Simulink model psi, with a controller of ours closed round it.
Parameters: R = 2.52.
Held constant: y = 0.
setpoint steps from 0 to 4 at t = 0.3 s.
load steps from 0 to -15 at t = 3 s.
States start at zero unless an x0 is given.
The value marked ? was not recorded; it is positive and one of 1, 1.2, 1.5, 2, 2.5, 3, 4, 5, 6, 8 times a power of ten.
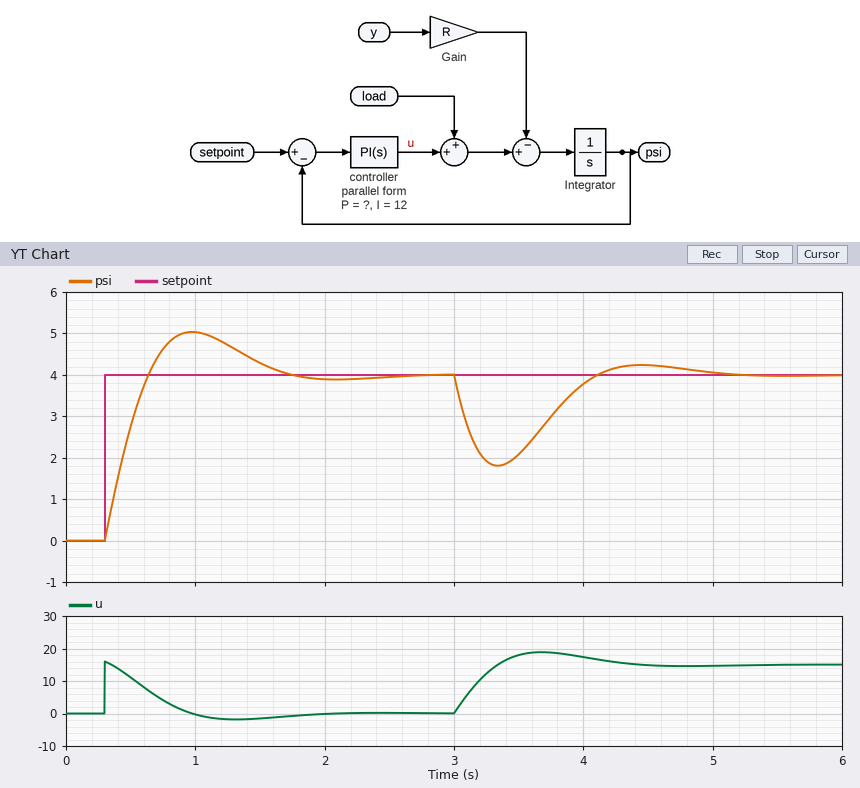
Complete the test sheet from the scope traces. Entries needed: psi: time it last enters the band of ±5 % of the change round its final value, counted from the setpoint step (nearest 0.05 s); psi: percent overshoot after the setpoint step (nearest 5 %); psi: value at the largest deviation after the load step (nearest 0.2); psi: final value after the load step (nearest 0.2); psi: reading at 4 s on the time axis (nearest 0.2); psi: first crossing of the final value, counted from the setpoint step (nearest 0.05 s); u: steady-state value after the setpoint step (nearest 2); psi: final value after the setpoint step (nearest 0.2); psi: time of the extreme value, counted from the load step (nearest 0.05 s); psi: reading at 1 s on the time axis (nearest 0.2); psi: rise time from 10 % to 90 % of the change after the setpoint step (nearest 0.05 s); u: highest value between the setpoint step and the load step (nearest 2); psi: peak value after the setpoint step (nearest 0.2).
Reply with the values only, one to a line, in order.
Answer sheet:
1.25 s
25 %
1.8
4.0
3.8
0.35 s
0
4.0
0.35 s
5.0
0.25 s
16
5.0
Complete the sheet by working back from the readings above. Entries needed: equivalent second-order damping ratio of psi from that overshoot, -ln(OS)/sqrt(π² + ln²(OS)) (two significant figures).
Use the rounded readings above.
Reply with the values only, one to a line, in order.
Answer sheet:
0.40
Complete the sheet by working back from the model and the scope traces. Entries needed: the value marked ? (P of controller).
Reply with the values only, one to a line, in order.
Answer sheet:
4
